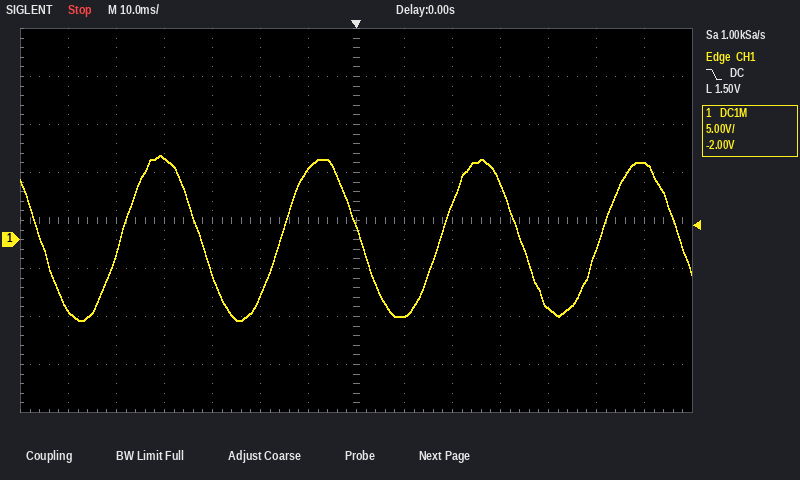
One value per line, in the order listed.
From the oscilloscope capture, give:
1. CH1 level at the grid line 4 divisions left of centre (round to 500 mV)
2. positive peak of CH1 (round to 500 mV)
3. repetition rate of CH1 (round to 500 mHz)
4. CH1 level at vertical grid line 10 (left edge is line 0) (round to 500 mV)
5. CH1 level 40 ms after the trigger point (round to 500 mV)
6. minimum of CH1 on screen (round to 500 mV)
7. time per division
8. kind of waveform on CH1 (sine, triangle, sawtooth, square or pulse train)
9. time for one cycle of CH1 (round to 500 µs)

8.5 V
9.0 V
30.0 Hz
6.0 V
-7.0 V
-8.5 V
10 ms
sine
33.5 ms
